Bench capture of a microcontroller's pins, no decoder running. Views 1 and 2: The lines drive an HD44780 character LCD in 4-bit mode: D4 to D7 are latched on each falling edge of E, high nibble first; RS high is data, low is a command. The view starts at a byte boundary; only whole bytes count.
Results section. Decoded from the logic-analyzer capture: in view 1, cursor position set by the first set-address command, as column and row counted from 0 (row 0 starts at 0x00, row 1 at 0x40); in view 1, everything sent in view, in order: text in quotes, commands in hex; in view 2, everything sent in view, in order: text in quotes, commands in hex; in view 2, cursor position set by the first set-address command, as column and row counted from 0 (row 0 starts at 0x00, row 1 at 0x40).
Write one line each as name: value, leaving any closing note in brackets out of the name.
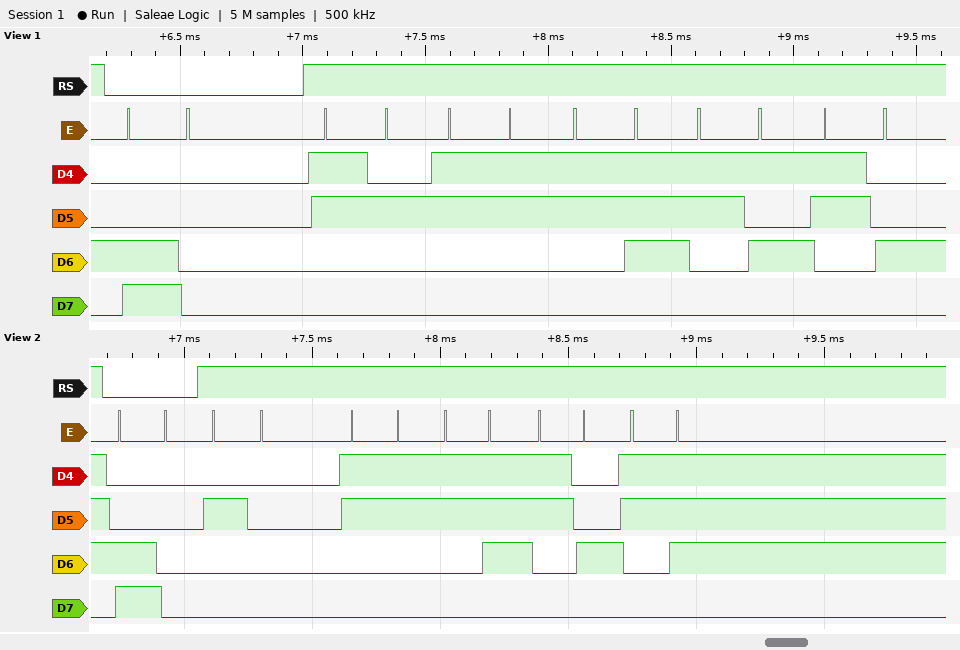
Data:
in view 1, cursor position set by the first set-address command, as column and row counted from 0: column 0, row 1
in view 1, everything sent in view, in order: text in quotes, commands in hex: 0xC0 "23754"
in view 2, everything sent in view, in order: text in quotes, commands in hex: 0xC0 " 3747"
in view 2, cursor position set by the first set-address command, as column and row counted from 0: column 0, row 1
